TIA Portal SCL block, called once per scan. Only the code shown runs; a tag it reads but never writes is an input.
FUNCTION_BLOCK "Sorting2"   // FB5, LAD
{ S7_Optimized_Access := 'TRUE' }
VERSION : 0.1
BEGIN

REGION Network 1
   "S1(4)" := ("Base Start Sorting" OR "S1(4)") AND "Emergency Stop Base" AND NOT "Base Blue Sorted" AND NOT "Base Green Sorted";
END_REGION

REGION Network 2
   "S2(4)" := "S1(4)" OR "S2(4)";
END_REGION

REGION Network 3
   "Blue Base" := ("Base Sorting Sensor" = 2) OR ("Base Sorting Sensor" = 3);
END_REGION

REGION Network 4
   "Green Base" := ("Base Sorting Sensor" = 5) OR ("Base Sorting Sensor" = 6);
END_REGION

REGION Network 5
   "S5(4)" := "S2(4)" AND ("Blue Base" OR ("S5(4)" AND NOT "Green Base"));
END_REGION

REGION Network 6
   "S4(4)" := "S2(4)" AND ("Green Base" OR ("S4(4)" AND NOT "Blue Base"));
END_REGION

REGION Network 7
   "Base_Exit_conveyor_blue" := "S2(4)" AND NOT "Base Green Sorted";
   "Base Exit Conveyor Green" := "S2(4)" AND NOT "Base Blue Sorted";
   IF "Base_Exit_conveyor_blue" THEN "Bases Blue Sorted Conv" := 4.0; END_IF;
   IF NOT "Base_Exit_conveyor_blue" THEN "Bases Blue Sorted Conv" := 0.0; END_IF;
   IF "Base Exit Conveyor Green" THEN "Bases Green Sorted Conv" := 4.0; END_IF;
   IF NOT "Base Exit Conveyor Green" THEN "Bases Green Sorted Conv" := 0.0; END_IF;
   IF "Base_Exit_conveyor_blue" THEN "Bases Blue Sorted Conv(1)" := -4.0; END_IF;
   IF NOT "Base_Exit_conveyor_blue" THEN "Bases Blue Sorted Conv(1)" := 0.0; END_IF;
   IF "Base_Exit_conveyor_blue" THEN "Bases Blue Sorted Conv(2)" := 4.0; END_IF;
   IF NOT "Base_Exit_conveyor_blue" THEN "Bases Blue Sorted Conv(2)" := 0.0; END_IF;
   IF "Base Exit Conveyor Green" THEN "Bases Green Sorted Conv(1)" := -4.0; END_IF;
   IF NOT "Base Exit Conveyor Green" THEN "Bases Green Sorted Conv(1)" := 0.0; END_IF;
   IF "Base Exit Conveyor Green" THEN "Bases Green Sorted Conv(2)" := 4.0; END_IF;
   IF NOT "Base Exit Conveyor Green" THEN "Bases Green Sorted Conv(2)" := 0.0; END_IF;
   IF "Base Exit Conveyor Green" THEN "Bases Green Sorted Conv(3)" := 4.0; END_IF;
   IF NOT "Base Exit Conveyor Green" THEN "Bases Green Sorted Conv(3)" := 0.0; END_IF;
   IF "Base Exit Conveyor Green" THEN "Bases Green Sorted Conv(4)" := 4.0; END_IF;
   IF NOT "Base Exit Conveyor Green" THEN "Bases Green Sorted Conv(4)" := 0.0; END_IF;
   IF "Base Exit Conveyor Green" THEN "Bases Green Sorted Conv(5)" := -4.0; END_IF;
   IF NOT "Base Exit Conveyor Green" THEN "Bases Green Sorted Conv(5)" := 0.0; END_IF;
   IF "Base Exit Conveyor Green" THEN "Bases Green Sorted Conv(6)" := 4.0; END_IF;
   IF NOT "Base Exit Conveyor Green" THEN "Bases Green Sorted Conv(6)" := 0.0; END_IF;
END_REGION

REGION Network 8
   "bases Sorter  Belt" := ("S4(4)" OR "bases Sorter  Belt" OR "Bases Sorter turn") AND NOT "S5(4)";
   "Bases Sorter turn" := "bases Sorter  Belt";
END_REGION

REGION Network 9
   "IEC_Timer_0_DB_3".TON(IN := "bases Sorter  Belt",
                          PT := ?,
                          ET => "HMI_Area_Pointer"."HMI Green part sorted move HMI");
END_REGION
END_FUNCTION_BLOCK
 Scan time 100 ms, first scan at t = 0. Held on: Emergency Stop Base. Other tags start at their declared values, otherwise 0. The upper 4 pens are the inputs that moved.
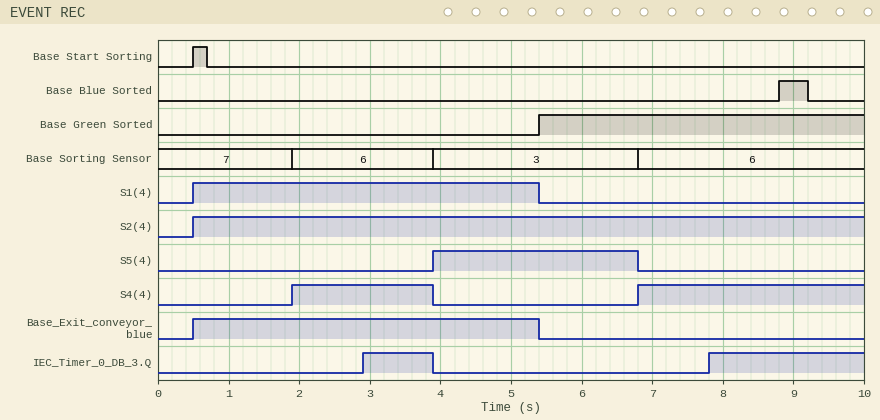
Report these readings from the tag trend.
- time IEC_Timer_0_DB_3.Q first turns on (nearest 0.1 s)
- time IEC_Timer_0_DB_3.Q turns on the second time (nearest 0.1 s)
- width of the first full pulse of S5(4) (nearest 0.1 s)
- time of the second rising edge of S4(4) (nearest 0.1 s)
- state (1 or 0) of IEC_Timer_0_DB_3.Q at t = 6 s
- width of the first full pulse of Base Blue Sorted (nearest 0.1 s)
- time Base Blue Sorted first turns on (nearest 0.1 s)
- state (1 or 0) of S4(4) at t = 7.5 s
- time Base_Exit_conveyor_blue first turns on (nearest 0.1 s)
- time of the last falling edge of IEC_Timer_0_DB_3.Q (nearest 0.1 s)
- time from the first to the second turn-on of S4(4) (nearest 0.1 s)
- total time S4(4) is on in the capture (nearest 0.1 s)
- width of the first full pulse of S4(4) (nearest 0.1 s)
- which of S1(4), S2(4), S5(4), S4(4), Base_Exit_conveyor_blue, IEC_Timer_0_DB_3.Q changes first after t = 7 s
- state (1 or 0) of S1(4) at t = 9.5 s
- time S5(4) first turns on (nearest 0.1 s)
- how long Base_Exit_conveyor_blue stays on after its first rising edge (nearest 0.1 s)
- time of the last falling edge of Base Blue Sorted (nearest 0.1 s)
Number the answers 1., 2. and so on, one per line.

1. 2.9 s
2. 7.8 s
3. 2.9 s
4. 6.8 s
5. 0
6. 0.4 s
7. 8.8 s
8. 1
9. 0.5 s
10. 3.9 s
11. 4.9 s
12. 5.2 s
13. 2.0 s
14. IEC_Timer_0_DB_3.Q
15. 0
16. 3.9 s
17. 4.9 s
18. 9.2 s
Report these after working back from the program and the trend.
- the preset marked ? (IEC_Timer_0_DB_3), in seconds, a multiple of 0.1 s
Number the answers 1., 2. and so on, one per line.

1. 1.0 s
